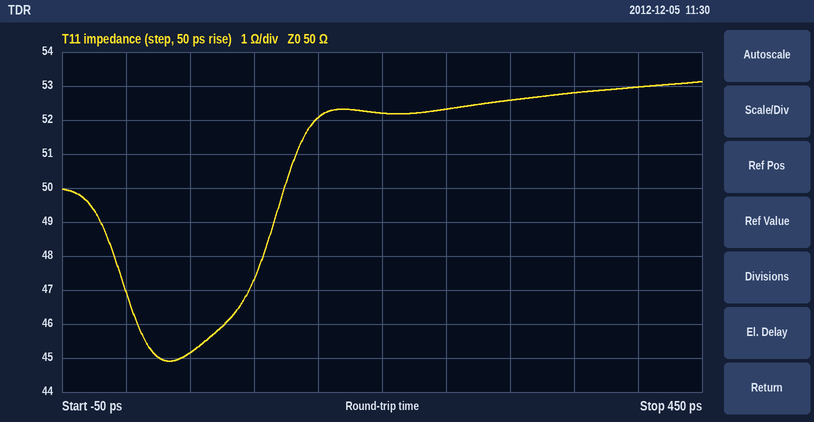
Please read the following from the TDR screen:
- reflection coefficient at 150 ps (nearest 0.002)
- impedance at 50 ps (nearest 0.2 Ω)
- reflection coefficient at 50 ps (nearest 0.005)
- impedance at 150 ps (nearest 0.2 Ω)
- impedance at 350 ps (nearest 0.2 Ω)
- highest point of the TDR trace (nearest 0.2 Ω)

+0.020
45.2 Ω
-0.050
52.0 Ω
52.8 Ω
53.2 Ω
